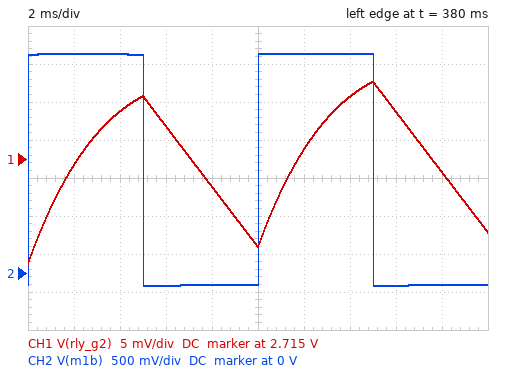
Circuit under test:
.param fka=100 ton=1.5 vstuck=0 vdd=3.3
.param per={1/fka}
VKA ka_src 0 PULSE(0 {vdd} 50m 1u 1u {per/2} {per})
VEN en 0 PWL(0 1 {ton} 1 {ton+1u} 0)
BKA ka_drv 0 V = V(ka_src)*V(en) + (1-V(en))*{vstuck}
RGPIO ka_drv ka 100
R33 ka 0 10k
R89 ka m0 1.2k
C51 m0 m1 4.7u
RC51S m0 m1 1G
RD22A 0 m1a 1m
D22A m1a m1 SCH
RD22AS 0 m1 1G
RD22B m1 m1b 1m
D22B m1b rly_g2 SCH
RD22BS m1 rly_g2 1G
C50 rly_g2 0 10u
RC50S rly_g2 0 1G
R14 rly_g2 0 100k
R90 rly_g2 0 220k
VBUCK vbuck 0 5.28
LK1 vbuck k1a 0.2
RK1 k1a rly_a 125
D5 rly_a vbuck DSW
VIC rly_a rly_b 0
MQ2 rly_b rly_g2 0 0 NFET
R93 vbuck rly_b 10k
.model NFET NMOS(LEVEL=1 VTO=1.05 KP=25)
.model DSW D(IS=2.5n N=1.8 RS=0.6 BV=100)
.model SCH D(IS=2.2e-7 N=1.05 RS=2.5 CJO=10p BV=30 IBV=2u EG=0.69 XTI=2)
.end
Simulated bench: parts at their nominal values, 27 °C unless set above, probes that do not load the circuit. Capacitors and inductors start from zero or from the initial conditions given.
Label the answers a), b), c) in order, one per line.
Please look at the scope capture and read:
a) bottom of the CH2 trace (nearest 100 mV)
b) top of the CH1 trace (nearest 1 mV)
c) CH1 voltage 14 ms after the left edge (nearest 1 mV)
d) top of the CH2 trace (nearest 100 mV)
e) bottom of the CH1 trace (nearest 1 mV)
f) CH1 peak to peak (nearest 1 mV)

a) -200 mV
b) 2.725 V
c) 2.723 V
d) 2.9 V
e) 2.701 V
f) 24 mV
